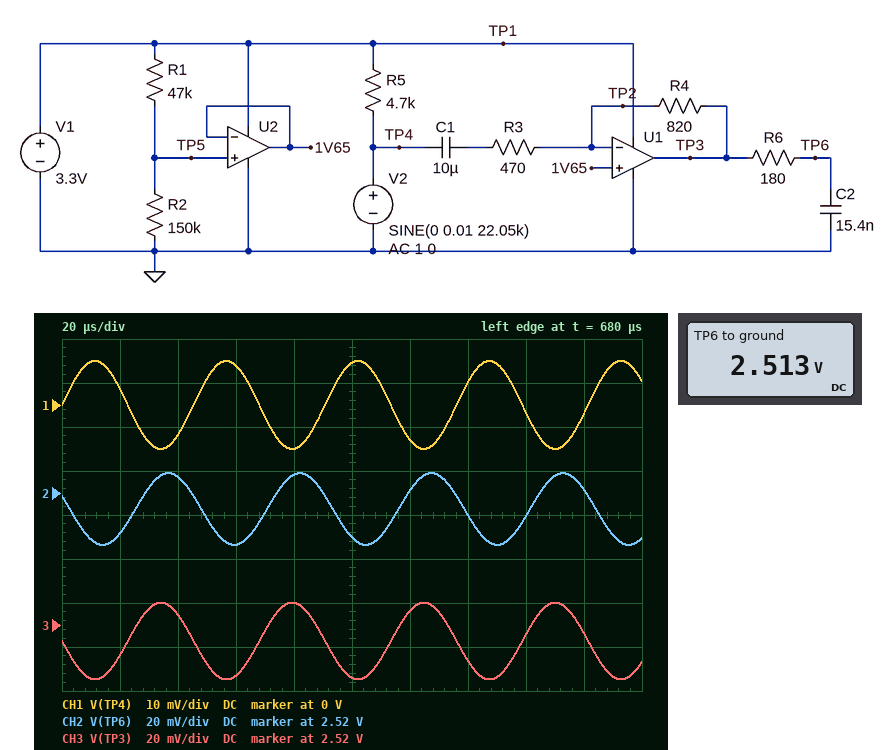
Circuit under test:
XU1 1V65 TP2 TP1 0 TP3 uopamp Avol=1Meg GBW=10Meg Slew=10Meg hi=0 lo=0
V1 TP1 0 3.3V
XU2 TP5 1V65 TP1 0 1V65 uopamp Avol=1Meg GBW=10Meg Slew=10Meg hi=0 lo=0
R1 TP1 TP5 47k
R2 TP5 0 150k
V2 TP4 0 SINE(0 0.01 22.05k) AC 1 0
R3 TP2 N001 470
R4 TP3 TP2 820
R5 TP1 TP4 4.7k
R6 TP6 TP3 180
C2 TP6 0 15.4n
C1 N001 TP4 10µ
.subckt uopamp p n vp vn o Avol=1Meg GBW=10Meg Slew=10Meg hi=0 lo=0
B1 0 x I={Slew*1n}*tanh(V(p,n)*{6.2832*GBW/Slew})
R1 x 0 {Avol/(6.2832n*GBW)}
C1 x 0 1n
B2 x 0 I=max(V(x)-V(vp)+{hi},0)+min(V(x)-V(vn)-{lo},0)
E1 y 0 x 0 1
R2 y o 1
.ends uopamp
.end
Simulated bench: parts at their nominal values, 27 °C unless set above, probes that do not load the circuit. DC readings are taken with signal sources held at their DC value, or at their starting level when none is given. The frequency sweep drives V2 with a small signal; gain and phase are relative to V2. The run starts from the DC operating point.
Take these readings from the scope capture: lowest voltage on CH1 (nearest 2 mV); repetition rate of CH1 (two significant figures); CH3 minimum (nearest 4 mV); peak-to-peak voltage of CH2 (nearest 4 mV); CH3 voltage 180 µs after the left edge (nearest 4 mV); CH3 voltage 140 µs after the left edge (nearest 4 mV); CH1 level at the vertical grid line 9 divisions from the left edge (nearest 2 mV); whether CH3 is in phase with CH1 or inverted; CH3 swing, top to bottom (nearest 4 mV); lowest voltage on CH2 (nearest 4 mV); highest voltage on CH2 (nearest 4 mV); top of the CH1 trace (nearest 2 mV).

-10 mV
22 kHz
2.496 V
32 mV
2.516 V
2.504 V
-2 mV
inverted
36 mV
2.496 V
2.528 V
10 mV
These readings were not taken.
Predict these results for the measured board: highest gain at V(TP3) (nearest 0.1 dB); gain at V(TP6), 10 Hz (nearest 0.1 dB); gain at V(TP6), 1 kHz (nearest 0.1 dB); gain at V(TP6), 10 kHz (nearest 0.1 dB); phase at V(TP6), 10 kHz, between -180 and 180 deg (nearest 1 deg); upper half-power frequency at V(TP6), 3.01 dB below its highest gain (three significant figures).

4.8 dB
-6.1 dB
4.8 dB
4.7 dB
170 deg
57.5 kHz
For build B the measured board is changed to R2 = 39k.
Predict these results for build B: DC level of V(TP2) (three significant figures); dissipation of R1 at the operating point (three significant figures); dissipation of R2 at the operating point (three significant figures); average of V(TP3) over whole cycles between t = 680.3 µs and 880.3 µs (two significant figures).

1.50 V
69.2 µW
57.4 µW
1.5 V
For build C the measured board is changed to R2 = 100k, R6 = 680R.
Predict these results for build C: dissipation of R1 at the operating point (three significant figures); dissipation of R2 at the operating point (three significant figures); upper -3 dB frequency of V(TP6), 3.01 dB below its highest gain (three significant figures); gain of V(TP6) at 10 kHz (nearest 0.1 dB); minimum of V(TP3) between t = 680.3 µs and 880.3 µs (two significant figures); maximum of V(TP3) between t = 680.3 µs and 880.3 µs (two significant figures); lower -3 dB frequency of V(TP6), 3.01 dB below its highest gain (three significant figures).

23.7 µW
50.4 µW
15.3 kHz
3.3 dB
2.2 V
2.3 V
33.7 Hz
